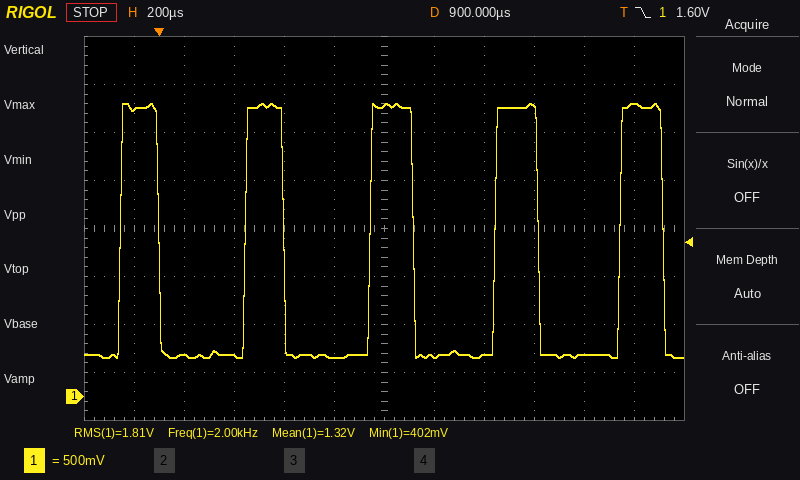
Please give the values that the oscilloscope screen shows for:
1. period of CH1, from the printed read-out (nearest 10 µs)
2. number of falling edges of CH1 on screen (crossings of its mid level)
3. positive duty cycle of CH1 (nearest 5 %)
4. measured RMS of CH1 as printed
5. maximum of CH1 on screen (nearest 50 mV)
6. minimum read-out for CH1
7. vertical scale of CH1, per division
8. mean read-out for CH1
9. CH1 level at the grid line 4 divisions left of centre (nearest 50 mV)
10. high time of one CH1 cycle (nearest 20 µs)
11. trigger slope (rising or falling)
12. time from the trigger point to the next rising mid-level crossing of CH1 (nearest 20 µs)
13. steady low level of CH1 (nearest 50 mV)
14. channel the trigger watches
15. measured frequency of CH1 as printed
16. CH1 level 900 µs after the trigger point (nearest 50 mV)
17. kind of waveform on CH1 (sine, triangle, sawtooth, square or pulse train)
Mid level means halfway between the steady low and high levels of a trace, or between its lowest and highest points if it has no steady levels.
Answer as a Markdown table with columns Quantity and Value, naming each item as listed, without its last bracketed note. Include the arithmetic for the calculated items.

| Quantity | Value |
|---|---|
| period of CH1, from the printed read-out | 1 / 2.00 kHz ≈ 500 µs |
| number of falling edges of CH1 on screen | 5 |
| positive duty cycle of CH1 | 35 % |
| measured RMS of CH1 as printed | 1.81 V |
| maximum of CH1 on screen | 3.05 V |
| minimum read-out for CH1 | 402 mV |
| vertical scale of CH1, per division | 500 mV |
| mean read-out for CH1 | 1.32 V |
| CH1 level at the grid line 4 divisions left of centre | 450 mV |
| high time of one CH1 cycle | 160 µs |
| trigger slope | falling |
| time from the trigger point to the next rising mid-level crossing of CH1 | 340 µs |
| steady low level of CH1 | 450 mV |
| channel the trigger watches | CH1 |
| measured frequency of CH1 as printed | 2.00 kHz |
| CH1 level 900 µs after the trigger point | 3.05 V |
| kind of waveform on CH1 | pulse train |
